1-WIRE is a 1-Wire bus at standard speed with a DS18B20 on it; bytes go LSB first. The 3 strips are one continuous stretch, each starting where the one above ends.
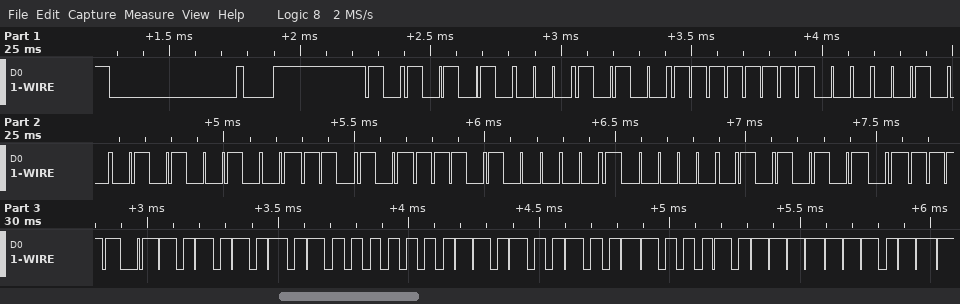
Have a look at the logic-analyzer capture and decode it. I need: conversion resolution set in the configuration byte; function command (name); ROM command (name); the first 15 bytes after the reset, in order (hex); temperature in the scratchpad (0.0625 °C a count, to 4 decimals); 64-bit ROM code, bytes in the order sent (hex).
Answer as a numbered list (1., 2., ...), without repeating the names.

1. 12 bits
2. Read Scratchpad
3. Match ROM
4. 55 28 FF 20 4A AE 17 04 AA BE 55 01 4B 46 7F
5. 21.3125 °C
6. 28 FF 20 4A AE 17 04 AA
